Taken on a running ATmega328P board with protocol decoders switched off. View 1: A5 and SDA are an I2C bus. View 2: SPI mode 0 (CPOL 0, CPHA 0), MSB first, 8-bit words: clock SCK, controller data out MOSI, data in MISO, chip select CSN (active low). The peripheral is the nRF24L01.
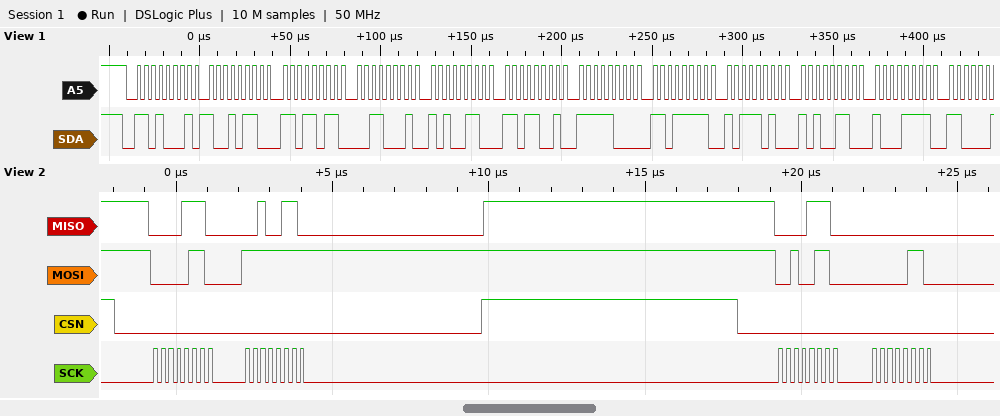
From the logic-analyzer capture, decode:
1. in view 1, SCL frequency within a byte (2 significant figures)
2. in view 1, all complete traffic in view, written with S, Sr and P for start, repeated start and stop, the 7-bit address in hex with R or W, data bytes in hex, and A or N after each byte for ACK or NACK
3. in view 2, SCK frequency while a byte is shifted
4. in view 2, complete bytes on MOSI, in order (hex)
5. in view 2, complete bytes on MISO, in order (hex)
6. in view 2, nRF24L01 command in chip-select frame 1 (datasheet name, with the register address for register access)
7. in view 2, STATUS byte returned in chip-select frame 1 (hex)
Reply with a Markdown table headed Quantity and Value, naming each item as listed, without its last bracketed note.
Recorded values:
| Quantity | Value |
|---|---|
| in view 1, SCL frequency within a byte | 250 kHz |
| in view 1, all complete traffic in view, written with S, Sr and P for start, repeated start and stop, the 7-bit address in hex with R or W, data bytes in hex, and A or N after each byte for ACK or NACK | S 68R A 96 A DB A 31 A A6 A D9 A F8 A DF A BA A A6 A 8F A |
| in view 2, SCK frequency while a byte is shifted | 4 MHz |
| in view 2, complete bytes on MOSI, in order | 06 FF 26 06 |
| in view 2, complete bytes on MISO, in order | 0E 26 0E 00 |
| in view 2, nRF24L01 command in chip-select frame 1 | R_REGISTER 0x06 |
| in view 2, STATUS byte returned in chip-select frame 1 | 0x0E |
